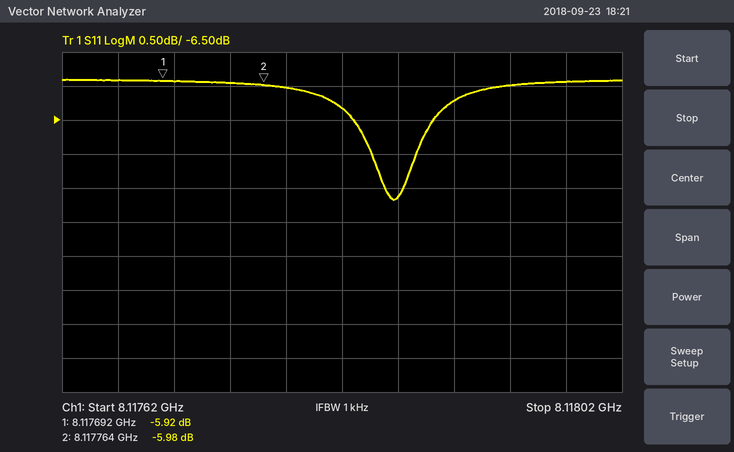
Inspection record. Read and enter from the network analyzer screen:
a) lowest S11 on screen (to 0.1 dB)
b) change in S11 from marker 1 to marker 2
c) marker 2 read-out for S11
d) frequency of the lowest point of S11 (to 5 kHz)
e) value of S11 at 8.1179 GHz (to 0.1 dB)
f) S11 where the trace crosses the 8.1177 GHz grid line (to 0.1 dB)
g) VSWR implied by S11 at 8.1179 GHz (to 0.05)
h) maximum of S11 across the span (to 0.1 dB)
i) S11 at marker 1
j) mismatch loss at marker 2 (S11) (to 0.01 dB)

-7.7 dB
-0.06 dB
-5.98 dB
8.117855 GHz
-6.2 dB
-5.9 dB
2.90
-5.9 dB
-5.92 dB
1.26 dB
